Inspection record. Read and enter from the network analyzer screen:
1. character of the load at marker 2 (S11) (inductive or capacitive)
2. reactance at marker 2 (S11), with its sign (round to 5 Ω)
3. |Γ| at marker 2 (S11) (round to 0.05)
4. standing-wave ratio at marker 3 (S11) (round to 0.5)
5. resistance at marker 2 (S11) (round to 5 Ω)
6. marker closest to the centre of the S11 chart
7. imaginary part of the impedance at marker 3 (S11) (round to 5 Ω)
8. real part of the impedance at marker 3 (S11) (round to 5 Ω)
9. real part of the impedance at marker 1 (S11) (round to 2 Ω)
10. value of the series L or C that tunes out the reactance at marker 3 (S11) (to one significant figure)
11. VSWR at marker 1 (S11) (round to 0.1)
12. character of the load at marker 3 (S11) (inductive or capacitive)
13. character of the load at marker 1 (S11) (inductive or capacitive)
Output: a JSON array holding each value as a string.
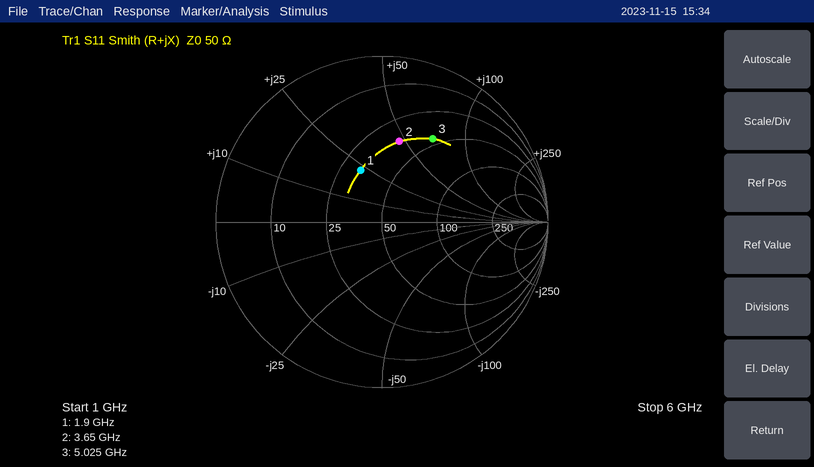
["inductive", "+45 Ω", "0.50", "4.0", "35 Ω", "marker 1", "+70 Ω", "45 Ω", "32 Ω", "500 fF", "2.0", "inductive", "inductive"]
